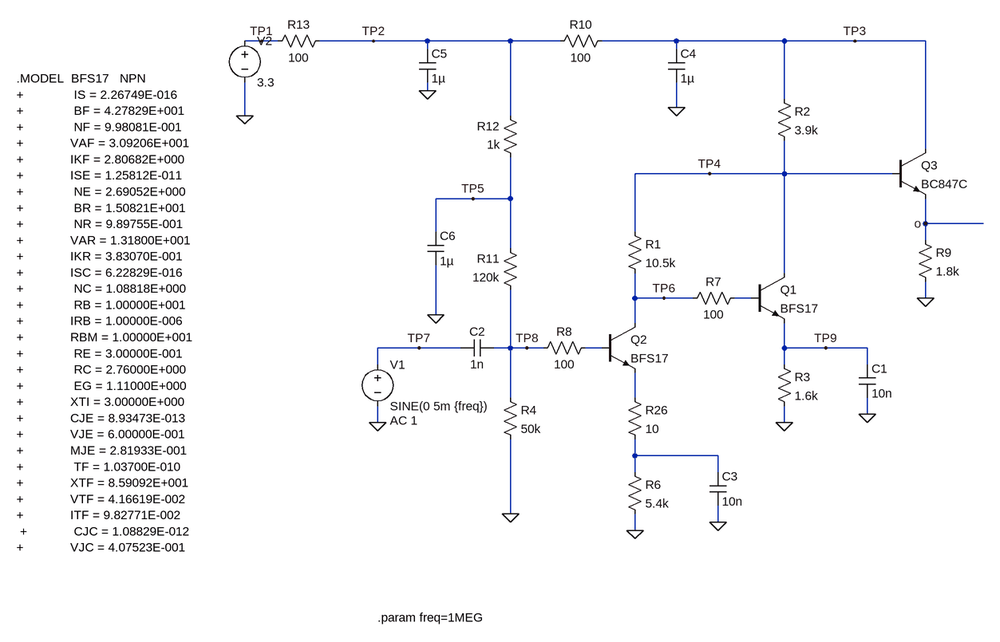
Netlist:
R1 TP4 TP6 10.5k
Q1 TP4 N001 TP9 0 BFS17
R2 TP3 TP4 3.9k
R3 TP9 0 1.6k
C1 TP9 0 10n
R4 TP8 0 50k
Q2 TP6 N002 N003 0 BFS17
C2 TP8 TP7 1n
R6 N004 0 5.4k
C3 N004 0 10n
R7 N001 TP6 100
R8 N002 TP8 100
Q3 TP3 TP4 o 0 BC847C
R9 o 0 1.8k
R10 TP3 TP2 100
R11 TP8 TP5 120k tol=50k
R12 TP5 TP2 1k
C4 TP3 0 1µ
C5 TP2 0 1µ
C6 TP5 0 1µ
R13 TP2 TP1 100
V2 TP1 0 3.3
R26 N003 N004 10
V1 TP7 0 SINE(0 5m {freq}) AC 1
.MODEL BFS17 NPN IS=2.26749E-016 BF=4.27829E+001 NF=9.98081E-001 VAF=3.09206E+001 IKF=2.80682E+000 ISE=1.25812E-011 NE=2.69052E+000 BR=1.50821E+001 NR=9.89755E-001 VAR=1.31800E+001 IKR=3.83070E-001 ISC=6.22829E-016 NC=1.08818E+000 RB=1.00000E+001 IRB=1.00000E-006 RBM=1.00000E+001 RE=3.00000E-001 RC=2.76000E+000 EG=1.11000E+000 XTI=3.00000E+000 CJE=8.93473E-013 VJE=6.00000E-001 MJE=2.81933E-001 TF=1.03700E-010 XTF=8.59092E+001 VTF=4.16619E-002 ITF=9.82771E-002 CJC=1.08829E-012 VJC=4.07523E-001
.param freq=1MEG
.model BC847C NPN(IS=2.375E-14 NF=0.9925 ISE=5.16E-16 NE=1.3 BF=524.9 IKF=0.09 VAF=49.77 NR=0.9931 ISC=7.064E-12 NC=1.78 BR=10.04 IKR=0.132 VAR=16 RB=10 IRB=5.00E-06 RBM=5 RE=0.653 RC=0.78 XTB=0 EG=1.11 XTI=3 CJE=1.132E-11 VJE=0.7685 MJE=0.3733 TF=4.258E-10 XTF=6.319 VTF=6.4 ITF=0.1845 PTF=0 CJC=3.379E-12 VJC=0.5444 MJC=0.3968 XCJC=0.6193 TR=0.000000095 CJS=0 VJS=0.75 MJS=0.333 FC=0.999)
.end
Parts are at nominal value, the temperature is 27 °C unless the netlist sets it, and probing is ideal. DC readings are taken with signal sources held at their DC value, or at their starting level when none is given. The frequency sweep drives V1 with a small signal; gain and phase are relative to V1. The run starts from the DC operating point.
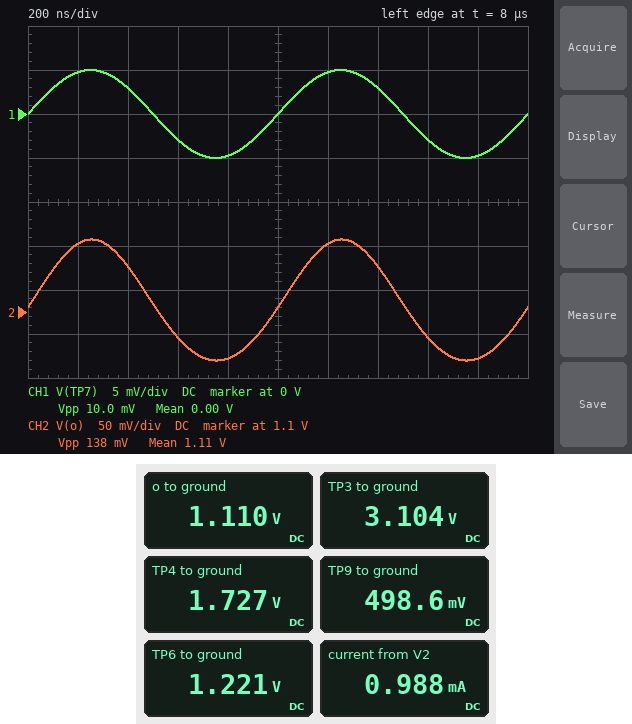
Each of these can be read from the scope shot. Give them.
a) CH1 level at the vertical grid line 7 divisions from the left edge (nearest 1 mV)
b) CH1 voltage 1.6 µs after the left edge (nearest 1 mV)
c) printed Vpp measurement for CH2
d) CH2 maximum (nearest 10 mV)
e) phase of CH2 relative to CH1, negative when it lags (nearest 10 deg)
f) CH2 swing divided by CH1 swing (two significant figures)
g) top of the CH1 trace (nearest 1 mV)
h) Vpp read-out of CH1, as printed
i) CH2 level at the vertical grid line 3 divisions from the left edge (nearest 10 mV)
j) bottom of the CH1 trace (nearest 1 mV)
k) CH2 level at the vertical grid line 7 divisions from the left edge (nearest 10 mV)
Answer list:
3 mV
-3 mV
138 mV
1.18 V
0 deg
14
5 mV
10.0 mV
1.07 V
-5 mV
1.15 V
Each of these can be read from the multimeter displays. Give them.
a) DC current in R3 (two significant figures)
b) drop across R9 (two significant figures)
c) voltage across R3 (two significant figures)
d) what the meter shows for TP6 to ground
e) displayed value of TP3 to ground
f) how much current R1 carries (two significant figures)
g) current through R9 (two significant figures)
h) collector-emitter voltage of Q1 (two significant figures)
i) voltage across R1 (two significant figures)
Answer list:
310 µA
1.1 V
500 mV
1.221 V
3.104 V
48 µA
620 µA
1.2 V
510 mV
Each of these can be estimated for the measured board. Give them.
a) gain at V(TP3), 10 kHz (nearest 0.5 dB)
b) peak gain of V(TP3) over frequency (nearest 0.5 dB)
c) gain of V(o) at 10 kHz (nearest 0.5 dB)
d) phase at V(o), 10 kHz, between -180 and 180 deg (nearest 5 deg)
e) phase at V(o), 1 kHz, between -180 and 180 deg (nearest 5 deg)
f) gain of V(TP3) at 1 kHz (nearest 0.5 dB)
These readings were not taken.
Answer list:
-38.0 dB
-37.0 dB
9.0 dB
95 deg
95 deg
-45.5 dB
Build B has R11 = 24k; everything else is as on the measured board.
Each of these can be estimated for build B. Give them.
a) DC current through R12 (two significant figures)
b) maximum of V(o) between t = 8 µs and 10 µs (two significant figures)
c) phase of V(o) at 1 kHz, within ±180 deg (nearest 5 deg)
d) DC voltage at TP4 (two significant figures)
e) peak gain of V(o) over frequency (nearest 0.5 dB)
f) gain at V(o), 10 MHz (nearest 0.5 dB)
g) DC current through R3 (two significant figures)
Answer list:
65 µA
1.6 V
-95 deg
2.2 V
15.5 dB
12.0 dB
110 µA
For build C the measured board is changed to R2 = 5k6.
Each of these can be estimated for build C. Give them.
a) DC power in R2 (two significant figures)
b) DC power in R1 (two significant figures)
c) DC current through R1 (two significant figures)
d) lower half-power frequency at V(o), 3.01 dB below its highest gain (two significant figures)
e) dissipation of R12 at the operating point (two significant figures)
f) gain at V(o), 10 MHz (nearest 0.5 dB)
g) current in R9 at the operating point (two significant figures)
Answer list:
430 µW
23 µW
47 µA
37 kHz
370 nW
22.0 dB
540 µA
